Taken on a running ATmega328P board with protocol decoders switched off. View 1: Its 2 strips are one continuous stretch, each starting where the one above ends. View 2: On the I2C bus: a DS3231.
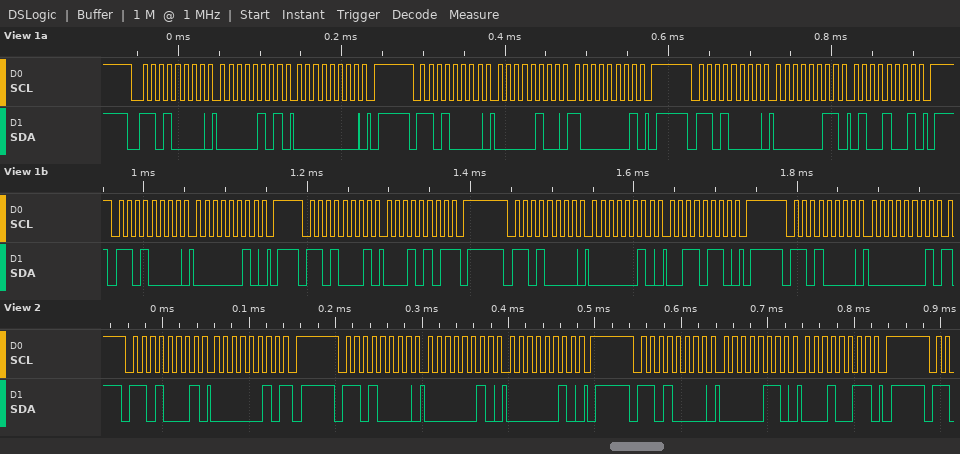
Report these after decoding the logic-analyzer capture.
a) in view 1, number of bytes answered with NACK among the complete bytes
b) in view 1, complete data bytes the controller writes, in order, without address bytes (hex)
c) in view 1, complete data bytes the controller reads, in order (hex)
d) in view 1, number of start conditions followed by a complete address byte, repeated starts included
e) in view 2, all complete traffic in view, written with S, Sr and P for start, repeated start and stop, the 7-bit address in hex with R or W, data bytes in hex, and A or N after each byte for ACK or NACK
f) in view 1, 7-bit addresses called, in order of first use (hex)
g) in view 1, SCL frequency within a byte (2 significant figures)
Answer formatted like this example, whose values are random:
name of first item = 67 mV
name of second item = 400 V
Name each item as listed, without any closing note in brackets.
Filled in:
in view 1, number of bytes answered with NACK among the complete bytes = 1
in view 1, complete data bytes the controller writes, in order, without address bytes = 05 00 04 81 03 49 02 02 36 01
in view 1, complete data bytes the controller reads, in order = 15
in view 1, number of start conditions followed by a complete address byte, repeated starts included = 7
in view 2, all complete traffic in view, written with S, Sr and P for start, repeated start and stop, the 7-bit address in hex with R or W, data bytes in hex, and A or N after each byte for ACK or NACK = S 68R A 02 N P S 68W A 02 A 02 A P S 68W A 06 A 13 A P
in view 1, 7-bit addresses called, in order of first use = 0x68
in view 1, SCL frequency within a byte = 100 kHz
